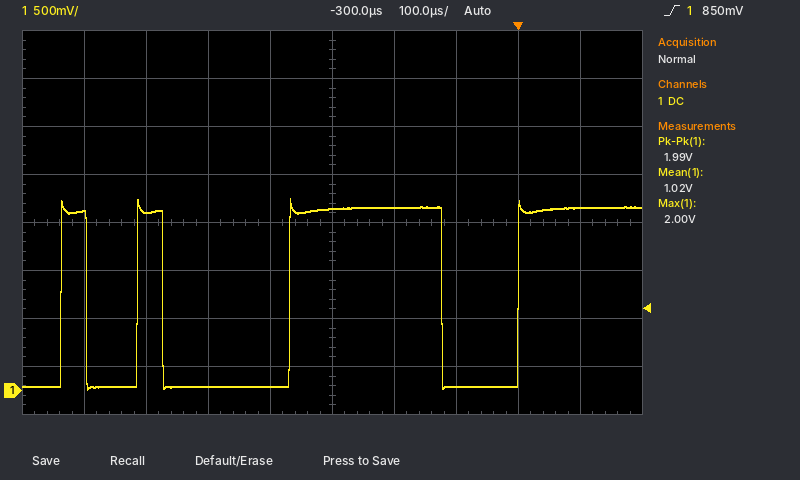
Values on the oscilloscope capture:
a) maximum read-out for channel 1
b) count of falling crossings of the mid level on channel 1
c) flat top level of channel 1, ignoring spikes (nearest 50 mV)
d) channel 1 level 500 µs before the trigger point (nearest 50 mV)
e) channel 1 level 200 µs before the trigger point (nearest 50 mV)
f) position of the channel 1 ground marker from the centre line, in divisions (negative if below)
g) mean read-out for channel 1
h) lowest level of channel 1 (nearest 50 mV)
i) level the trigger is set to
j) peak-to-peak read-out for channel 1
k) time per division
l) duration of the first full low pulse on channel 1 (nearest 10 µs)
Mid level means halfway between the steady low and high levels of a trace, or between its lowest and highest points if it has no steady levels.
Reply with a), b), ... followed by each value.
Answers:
a) 2.00 V
b) 3
c) 1.90 V
d) 50 mV
e) 1.90 V
f) -3.5 div
g) 1.02 V
h) 0 mV
i) 850 mV
j) 1.99 V
k) 100 µs
l) 80 µs
